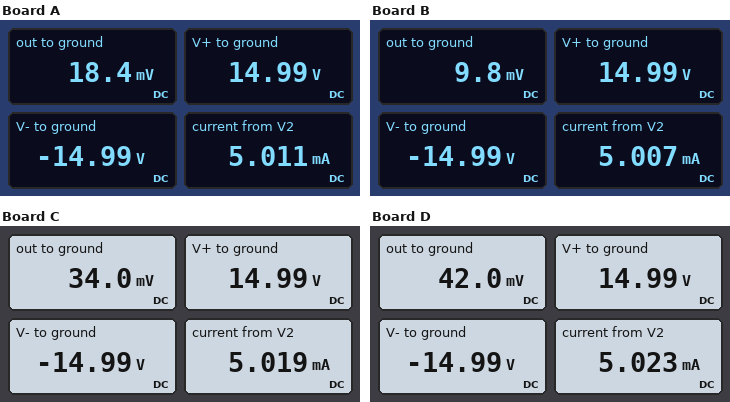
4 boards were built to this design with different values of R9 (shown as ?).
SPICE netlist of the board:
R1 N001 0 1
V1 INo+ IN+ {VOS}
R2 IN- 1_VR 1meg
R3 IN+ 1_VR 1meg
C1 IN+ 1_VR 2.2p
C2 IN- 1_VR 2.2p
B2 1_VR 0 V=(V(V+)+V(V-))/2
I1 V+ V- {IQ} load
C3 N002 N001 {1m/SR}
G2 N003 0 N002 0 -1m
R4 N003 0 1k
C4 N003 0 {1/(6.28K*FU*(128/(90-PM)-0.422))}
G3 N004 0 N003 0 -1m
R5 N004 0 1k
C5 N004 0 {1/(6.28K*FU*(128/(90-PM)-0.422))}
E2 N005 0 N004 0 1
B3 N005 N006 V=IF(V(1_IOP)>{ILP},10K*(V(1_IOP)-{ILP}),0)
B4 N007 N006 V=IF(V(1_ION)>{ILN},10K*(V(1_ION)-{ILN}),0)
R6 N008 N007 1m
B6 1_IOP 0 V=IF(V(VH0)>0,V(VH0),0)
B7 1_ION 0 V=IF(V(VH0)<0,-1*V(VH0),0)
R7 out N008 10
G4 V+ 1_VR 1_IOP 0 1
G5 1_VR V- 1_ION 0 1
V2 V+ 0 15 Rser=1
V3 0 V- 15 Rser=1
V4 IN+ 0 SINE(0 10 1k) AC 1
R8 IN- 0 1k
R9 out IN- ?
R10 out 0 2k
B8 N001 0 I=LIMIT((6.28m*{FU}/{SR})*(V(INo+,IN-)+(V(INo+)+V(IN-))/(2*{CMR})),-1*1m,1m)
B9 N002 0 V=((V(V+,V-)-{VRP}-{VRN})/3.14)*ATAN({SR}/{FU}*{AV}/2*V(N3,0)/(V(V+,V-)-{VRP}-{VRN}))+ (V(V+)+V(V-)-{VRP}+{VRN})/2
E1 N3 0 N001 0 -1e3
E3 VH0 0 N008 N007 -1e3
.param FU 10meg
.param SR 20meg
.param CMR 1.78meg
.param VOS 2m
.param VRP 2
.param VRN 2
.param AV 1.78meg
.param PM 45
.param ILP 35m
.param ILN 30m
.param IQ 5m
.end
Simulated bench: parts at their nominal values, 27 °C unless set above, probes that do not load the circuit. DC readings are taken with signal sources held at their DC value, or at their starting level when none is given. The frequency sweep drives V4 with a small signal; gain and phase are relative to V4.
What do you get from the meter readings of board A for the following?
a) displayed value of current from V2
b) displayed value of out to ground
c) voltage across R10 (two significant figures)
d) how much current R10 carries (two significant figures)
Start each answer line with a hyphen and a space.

- 5.011 mA
- 18.4 mV
- 18 mV
- 9.2 µA
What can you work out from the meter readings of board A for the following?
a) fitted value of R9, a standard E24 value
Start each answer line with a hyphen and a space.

- 8.2 kΩ
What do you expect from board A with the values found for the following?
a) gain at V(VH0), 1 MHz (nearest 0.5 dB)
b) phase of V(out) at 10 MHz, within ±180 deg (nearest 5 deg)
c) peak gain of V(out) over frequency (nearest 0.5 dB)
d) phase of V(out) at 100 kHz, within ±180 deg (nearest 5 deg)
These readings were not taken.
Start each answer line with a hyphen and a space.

- -47.5 dB
- -130 deg
- 19.5 dB
- -5 deg
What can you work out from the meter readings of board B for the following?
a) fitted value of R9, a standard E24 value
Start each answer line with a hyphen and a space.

- 3.9 kΩ
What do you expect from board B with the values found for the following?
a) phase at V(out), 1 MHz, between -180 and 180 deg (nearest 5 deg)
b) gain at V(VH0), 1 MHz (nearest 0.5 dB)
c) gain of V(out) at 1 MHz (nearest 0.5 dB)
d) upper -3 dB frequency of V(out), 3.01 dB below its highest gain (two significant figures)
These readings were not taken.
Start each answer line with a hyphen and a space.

- -25 deg
- -50.0 dB
- 13.0 dB
- 2.5 MHz
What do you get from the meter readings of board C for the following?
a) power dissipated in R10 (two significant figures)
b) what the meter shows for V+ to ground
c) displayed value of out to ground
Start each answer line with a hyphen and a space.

- 580 nW
- 14.99 V
- 34.0 mV
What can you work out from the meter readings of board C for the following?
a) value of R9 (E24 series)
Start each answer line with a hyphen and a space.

- 16 kΩ
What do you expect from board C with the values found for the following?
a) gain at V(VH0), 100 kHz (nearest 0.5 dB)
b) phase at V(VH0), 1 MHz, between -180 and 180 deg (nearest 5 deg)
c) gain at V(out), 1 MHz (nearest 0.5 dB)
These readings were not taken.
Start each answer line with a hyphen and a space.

- -40.5 dB
- -65 deg
- 19.0 dB
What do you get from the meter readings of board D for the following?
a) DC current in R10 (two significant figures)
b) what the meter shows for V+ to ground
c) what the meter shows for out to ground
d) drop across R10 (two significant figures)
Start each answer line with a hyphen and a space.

- 21 µA
- 14.99 V
- 42.0 mV
- 42 mV
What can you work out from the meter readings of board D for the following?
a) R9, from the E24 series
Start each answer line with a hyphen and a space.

- 20 kΩ
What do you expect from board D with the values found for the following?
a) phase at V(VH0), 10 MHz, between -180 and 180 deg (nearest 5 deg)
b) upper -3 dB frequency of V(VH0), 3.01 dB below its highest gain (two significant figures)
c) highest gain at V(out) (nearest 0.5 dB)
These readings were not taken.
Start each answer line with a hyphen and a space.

- -135 deg
- 500 kHz
- 26.5 dB
